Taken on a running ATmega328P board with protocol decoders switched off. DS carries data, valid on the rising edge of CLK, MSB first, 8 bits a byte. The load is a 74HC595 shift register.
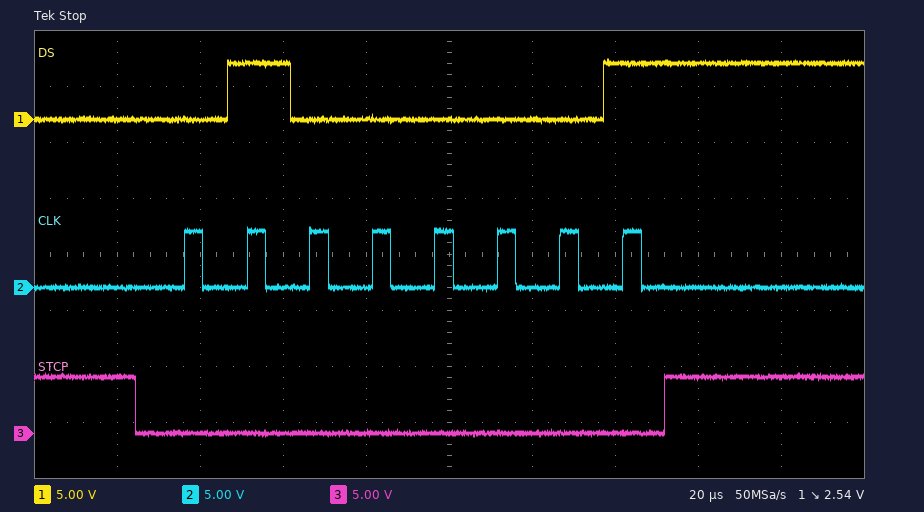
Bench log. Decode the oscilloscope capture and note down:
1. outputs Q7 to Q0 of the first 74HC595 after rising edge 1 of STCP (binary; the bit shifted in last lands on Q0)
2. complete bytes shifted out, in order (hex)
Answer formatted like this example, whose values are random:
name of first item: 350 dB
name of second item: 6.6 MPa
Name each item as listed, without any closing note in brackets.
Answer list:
outputs Q7 to Q0 of the first 74HC595 after rising edge 1 of STCP: 01000001
complete bytes shifted out, in order: 41
